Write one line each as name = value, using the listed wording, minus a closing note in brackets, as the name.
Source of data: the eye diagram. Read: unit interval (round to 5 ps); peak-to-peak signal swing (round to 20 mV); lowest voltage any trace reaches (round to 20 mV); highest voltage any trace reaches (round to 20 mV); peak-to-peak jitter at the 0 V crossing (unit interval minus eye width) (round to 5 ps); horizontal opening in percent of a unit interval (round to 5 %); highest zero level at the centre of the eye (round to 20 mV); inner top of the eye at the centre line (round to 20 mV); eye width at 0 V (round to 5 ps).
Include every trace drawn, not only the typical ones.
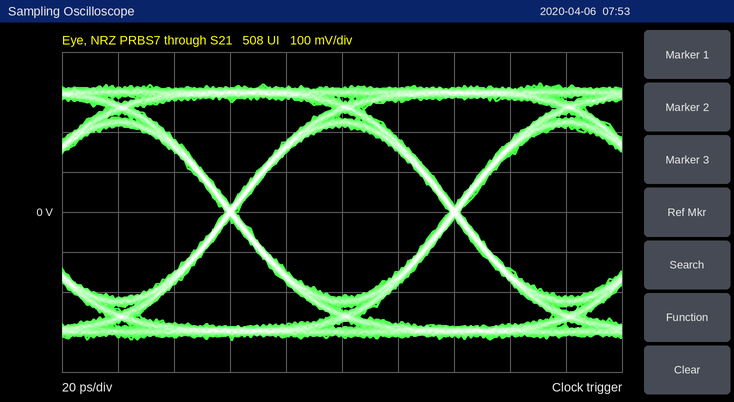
unit interval = 80 ps
peak-to-peak signal swing = 640 mV
lowest voltage any trace reaches = -320 mV
highest voltage any trace reaches = 320 mV
peak-to-peak jitter at the 0 V crossing (unit interval minus eye width) = 5 ps
horizontal opening in percent of a unit interval = 95 %
highest zero level at the centre of the eye = -220 mV
inner top of the eye at the centre line = 220 mV
eye width at 0 V = 75 ps
